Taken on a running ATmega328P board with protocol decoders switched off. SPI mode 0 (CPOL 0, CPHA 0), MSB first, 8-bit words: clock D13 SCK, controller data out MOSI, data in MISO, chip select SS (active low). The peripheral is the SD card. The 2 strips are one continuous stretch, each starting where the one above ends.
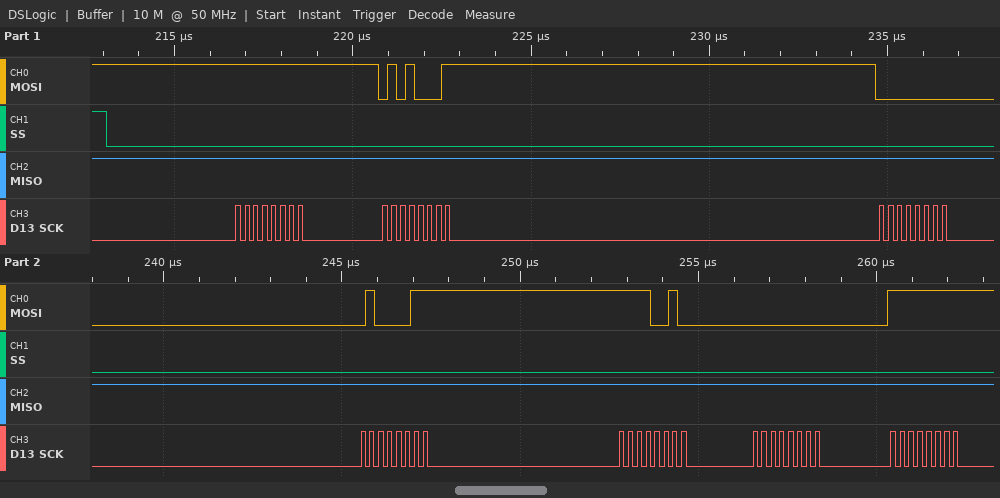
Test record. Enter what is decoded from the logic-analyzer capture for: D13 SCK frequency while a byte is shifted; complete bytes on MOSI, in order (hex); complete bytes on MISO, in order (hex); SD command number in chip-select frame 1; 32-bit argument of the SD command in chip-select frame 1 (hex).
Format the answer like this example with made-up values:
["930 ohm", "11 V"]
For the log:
["4 MHz", "FF 51 00 43 F2 00 FF", "FF FF FF FF FF FF FF", "CMD17", "0x0043F200"]
